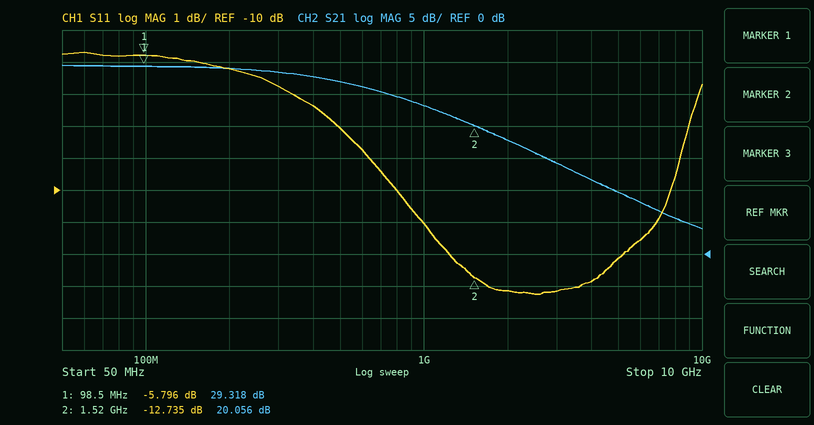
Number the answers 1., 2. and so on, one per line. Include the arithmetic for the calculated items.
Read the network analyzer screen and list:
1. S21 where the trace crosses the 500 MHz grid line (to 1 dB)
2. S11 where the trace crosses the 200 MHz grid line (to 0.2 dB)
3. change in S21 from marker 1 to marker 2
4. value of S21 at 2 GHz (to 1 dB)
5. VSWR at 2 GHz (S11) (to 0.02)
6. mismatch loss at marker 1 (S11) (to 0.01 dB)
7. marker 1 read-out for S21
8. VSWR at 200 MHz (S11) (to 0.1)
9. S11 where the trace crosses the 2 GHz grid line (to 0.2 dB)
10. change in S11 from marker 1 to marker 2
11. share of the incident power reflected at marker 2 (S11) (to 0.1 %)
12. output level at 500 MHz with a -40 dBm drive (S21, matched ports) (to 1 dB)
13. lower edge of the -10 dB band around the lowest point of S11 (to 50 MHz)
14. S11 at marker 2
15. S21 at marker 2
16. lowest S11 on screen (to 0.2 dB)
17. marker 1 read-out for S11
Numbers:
1. 27 dB
2. -6.2 dB
3. 20.056 − (29.318) = -9.262 dB
4. 18 dB
5. |Γ| = 10^(-13.2/20) = 0.2188; VSWR = (1 + 0.2188)/(1 − 0.2188) ≈ 1.56
6. −10 log10(1 − 10^(-5.796/10)) ≈ 1.33 dB
7. 29.318 dB
8. |Γ| = 10^(-6.2/20) = 0.4898; VSWR = (1 + 0.4898)/(1 − 0.4898) ≈ 2.9
9. -13.2 dB
10. -12.735 − (-5.796) = -6.939 dB
11. 10^(-12.735/10) ≈ 5.3 %
12. -40 dBm + (27 dB) = -13 dBm
13. 800 MHz
14. -12.735 dB
15. 20.056 dB
16. -13.2 dB
17. -5.796 dB
